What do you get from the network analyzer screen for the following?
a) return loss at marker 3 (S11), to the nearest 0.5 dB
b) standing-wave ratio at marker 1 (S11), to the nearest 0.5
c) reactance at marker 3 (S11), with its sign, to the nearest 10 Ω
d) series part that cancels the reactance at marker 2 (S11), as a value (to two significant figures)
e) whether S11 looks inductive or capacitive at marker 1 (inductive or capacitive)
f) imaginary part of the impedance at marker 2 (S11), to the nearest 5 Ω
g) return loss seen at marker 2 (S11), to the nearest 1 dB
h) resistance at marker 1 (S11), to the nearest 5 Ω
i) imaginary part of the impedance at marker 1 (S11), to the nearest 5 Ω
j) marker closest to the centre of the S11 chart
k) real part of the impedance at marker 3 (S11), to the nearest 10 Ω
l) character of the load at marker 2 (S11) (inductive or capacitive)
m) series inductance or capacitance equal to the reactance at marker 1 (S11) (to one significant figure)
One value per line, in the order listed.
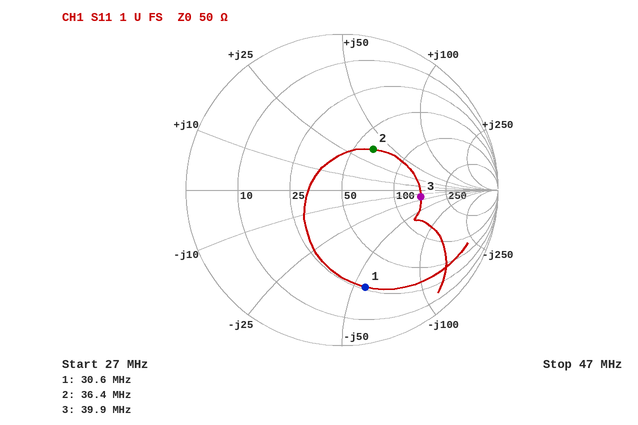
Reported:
6.0 dB
4.5
-20 Ω
120 pF
capacitive
+35 Ω
10 dB
25 Ω
-55 Ω
marker 2
150 Ω
inductive
90 pF
